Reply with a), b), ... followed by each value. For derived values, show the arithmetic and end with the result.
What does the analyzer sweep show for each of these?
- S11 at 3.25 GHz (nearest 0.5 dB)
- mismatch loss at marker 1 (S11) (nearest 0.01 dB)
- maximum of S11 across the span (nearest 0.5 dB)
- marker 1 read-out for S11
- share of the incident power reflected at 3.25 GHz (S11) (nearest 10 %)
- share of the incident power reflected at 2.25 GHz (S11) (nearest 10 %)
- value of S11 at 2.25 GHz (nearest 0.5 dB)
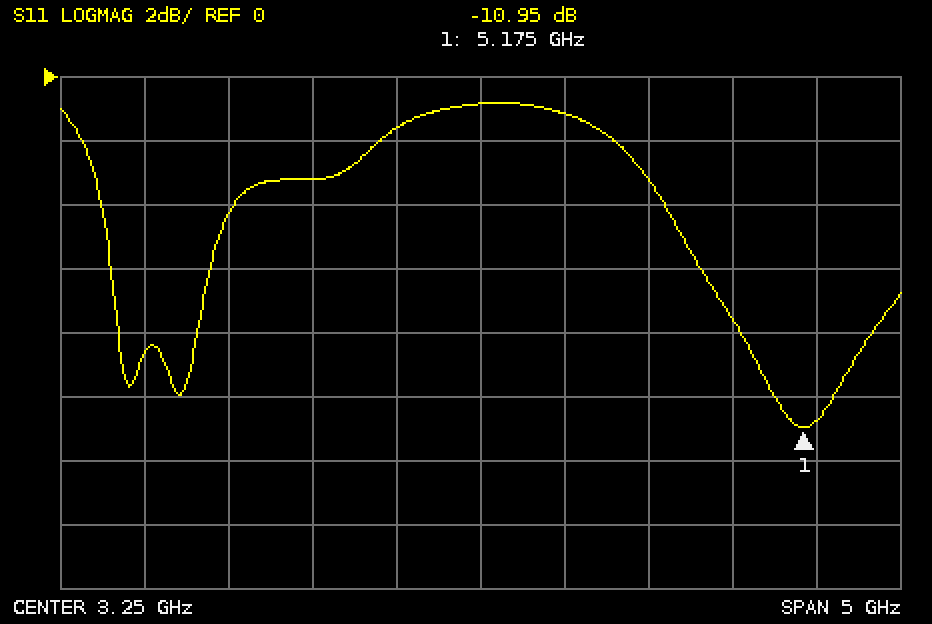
a) -1.0 dB
b) −10 log10(1 − 10^(-10.95/10)) ≈ 0.36 dB
c) -1.0 dB
d) -10.95 dB
e) 10^(-1/10) ≈ 79.4 %, so 80 % to the nearest 10 %
f) 10^(-3/10) ≈ 50 %
g) -3.0 dB
